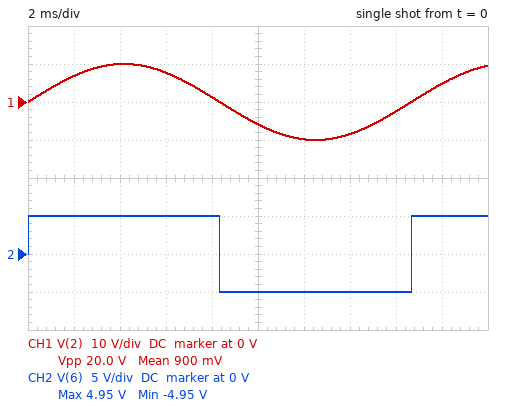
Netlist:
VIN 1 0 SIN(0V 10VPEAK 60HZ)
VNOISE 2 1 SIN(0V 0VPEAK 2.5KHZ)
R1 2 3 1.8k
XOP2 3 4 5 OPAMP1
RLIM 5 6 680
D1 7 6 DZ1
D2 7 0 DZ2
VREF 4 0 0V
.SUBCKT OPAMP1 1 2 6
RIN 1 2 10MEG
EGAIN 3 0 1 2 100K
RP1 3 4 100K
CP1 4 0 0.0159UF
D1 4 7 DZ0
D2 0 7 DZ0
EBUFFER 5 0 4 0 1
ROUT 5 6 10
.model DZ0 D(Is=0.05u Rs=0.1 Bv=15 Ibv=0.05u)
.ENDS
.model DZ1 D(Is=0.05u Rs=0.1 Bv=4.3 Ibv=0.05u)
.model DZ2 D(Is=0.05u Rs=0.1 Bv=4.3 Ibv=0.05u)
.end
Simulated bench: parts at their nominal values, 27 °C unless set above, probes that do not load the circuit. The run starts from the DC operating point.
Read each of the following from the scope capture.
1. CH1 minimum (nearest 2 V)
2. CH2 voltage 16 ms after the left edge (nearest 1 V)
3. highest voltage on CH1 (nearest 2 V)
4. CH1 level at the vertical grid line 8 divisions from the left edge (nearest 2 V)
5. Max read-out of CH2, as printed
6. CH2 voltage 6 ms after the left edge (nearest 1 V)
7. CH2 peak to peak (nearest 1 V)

-10 V
-5 V
10 V
-2 V
4.95 V
5 V
10 V
